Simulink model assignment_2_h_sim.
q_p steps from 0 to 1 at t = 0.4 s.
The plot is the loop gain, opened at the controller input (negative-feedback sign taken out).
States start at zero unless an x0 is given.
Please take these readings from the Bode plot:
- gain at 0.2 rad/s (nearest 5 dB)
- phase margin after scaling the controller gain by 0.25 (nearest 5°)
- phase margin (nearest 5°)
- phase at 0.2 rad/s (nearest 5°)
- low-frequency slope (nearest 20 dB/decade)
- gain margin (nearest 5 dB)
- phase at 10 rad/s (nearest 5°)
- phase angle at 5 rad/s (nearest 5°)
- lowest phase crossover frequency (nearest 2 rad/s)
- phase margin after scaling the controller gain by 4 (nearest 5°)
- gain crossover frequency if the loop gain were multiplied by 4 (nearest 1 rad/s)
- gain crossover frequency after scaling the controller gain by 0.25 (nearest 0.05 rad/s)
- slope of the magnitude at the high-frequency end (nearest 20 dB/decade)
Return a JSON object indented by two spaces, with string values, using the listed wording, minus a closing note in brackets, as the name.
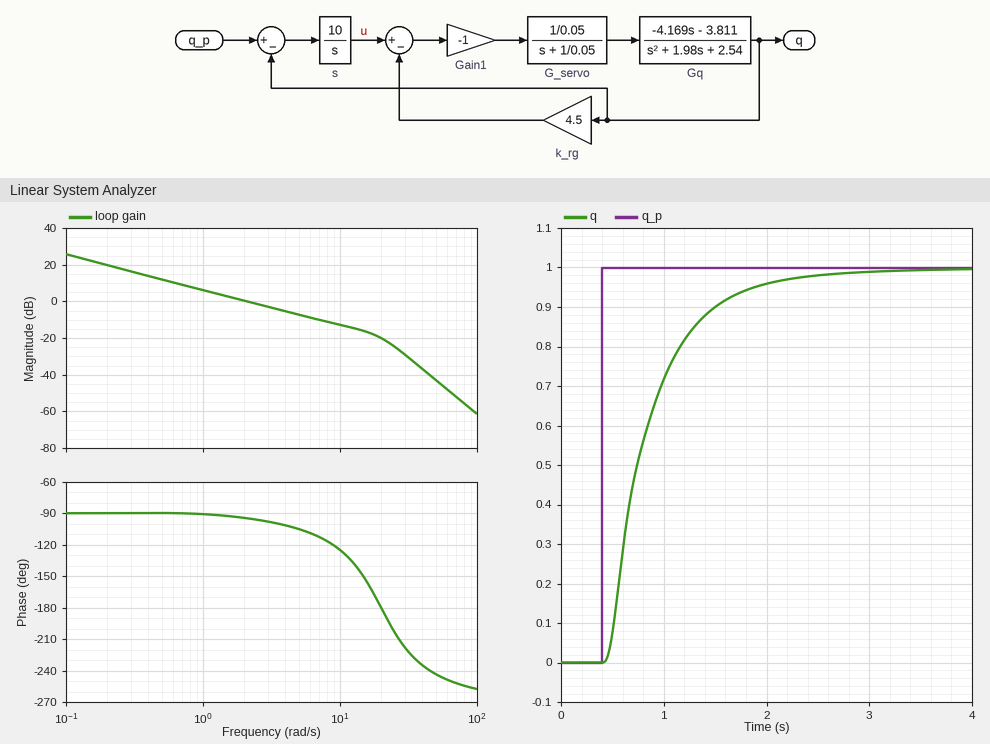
{
  "gain at 0.2 rad/s": "20 dB",
  "phase margin after scaling the controller gain by 0.25": "90°",
  "phase margin": "85°",
  "phase at 0.2 rad/s": "-90°",
  "low-frequency slope": "-20 dB/decade",
  "gain margin": "20 dB",
  "phase at 10 rad/s": "-125°",
  "phase angle at 5 rad/s": "-105°",
  "lowest phase crossover frequency": "20 rad/s",
  "phase margin after scaling the controller gain by 4": "60°",
  "gain crossover frequency if the loop gain were multiplied by 4": "9 rad/s",
  "gain crossover frequency after scaling the controller gain by 0.25": "0.50 rad/s",
  "slope of the magnitude at the high-frequency end": "-60 dB/decade"
}
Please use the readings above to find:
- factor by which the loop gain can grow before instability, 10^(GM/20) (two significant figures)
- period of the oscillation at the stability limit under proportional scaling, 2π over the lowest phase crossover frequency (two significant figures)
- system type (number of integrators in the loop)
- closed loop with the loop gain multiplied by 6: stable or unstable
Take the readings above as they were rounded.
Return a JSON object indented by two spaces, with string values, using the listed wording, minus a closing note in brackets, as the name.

{
  "factor by which the loop gain can grow before instability, 10^(GM/20)": "10",
  "period of the oscillation at the stability limit under proportional scaling, 2π over the lowest phase crossover frequency": "0.31 s",
  "system type": "1",
  "closed loop with the loop gain multiplied by 6: stable or unstable": "stable"
}
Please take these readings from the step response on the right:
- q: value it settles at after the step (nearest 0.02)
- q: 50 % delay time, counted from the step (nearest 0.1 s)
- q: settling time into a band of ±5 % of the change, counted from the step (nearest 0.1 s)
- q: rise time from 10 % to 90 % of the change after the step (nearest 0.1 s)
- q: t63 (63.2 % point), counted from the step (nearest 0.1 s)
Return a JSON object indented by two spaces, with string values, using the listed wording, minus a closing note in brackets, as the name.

{
  "q: value it settles at after the step": "1.00",
  "q: 50 % delay time, counted from the step": "0.3 s",
  "q: settling time into a band of ±5 % of the change, counted from the step": "1.5 s",
  "q: rise time from 10 % to 90 % of the change after the step": "1.0 s",
  "q: t63 (63.2 % point), counted from the step": "0.5 s"
}
